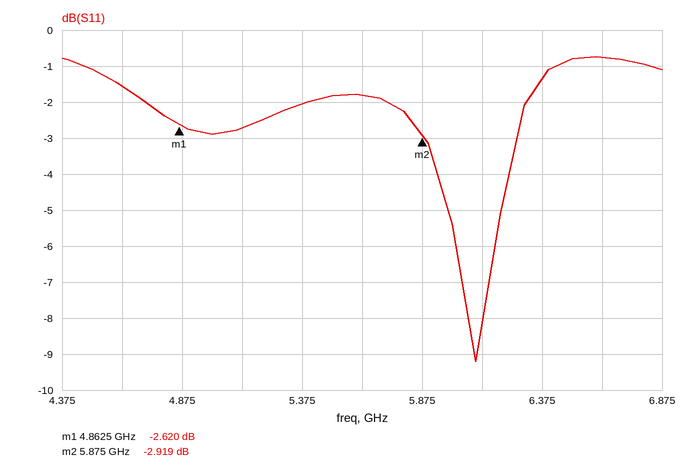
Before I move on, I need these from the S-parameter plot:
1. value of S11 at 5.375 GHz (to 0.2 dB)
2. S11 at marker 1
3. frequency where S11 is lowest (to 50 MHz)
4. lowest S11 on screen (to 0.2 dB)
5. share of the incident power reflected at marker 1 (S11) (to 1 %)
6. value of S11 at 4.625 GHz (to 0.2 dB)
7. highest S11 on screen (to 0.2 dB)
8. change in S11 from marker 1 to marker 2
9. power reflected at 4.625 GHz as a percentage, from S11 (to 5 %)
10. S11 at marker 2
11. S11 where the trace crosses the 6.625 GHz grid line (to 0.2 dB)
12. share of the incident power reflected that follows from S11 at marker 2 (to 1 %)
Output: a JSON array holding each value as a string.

["-2.0 dB", "-2.620 dB", "6.10 GHz", "-9.2 dB", "55 %", "-1.6 dB", "-0.8 dB", "-0.299 dB", "70 %", "-2.919 dB", "-0.8 dB", "51 %"]
